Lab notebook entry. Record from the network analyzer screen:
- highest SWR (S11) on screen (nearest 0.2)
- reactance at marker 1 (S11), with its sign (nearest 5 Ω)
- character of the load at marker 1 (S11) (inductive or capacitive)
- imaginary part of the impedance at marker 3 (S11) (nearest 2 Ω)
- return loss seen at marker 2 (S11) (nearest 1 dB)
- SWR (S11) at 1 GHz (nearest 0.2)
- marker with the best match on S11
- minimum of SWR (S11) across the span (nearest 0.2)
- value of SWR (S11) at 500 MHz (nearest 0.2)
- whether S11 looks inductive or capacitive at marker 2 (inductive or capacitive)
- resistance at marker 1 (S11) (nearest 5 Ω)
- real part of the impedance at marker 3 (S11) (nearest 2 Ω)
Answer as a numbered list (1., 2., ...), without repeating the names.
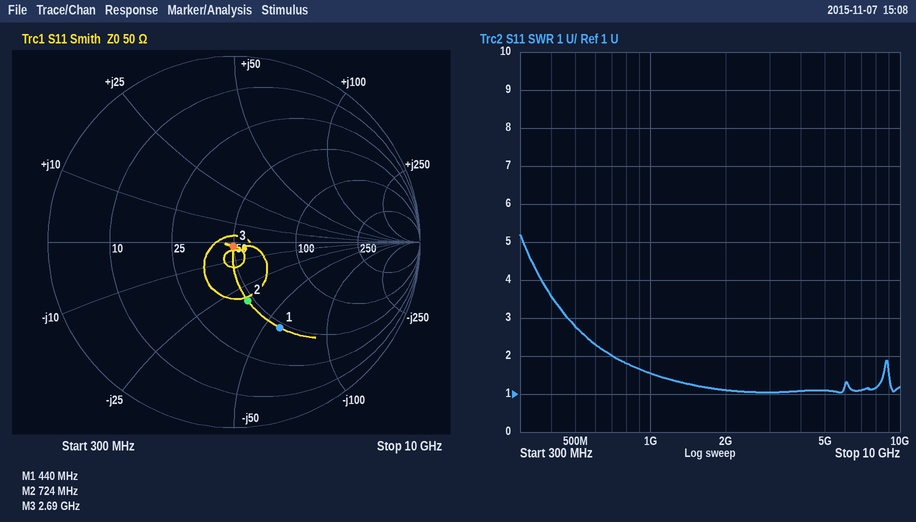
1. 5.2
2. -60 Ω
3. capacitive
4. -2 Ω
5. 10 dB
6. 1.6
7. marker 3
8. 1.0
9. 2.8
10. capacitive
11. 45 Ω
12. 50 Ω
